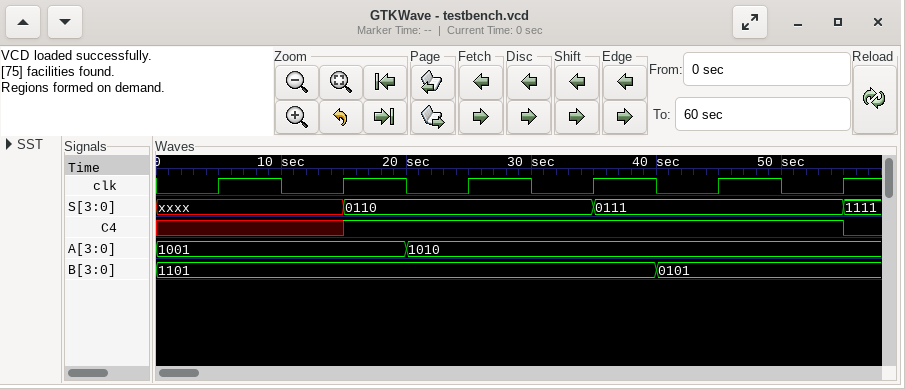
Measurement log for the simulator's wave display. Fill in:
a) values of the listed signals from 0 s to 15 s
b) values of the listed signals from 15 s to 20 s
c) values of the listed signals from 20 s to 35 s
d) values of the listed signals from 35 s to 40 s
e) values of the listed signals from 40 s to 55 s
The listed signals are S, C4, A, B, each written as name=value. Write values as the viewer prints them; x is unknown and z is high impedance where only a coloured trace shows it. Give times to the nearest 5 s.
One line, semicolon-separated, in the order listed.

S=xxxx, C4=x, A=1001, B=1101; S=0110, C4=1, A=1001, B=1101; S=0110, C4=1, A=1010, B=1101; S=0111, C4=1, A=1010, B=1101; S=0111, C4=1, A=1010, B=0101
